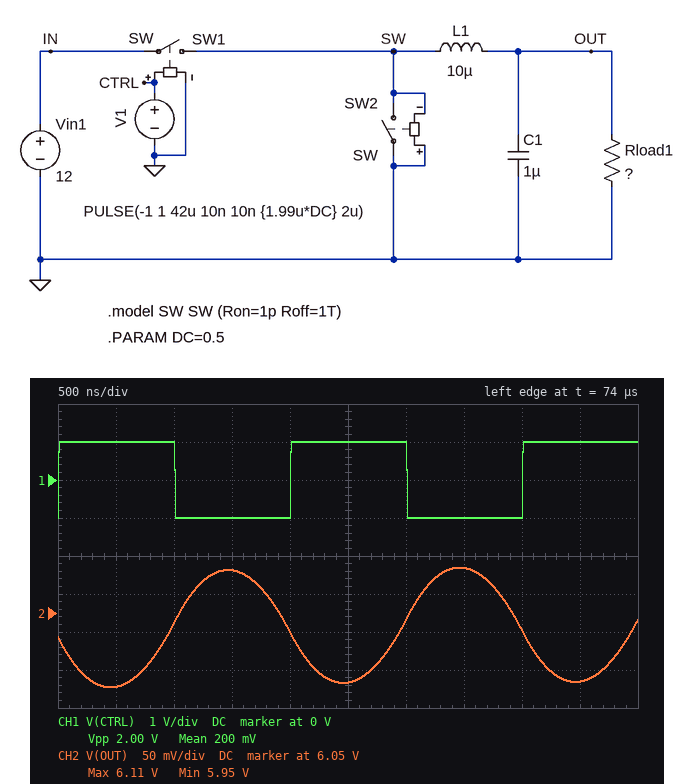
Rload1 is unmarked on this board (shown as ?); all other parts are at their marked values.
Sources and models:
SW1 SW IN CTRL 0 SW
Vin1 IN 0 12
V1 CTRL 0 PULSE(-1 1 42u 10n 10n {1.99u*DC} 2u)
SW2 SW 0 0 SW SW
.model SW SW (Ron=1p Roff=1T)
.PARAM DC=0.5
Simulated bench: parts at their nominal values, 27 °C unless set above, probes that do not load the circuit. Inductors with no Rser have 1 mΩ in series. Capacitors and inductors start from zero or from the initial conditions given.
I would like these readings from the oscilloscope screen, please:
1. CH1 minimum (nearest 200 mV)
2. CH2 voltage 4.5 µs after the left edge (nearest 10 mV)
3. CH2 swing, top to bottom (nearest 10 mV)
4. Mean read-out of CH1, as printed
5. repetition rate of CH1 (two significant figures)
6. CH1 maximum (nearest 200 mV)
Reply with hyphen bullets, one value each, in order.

- -1.0 V
- 5.96 V
- 160 mV
- 200 mV
- 500 kHz
- 1.0 V
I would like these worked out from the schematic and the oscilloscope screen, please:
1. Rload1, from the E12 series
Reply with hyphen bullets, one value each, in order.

- 2.7 Ω
